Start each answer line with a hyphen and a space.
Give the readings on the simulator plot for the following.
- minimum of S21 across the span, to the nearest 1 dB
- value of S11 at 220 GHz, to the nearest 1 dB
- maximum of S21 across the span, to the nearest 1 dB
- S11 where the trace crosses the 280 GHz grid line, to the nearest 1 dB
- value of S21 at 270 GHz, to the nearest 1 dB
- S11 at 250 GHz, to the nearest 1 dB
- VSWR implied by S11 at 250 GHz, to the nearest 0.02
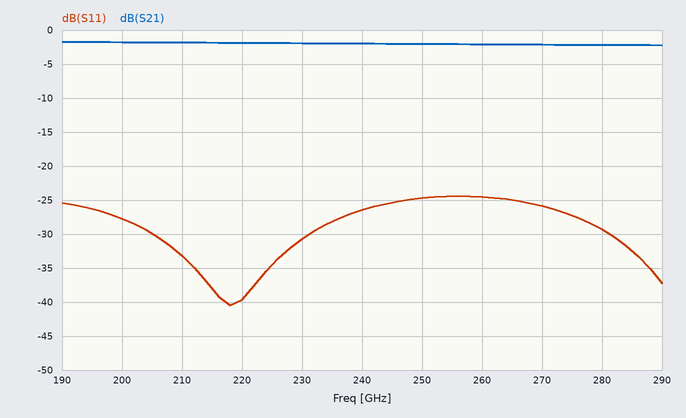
- -2 dB
- -40 dB
- -2 dB
- -29 dB
- -2 dB
- -25 dB
- 1.12
